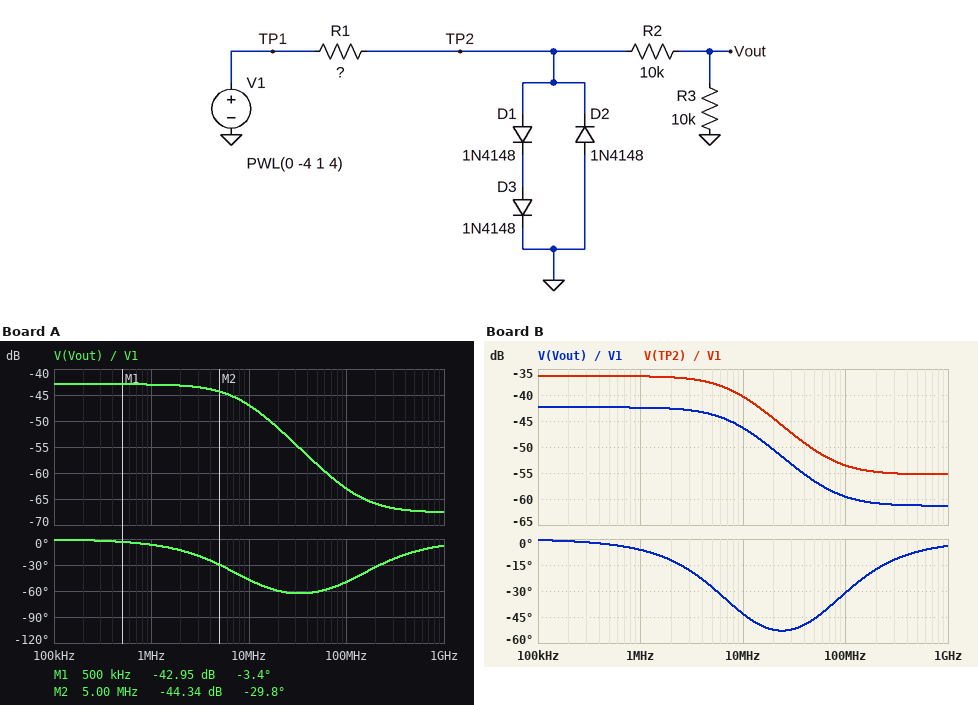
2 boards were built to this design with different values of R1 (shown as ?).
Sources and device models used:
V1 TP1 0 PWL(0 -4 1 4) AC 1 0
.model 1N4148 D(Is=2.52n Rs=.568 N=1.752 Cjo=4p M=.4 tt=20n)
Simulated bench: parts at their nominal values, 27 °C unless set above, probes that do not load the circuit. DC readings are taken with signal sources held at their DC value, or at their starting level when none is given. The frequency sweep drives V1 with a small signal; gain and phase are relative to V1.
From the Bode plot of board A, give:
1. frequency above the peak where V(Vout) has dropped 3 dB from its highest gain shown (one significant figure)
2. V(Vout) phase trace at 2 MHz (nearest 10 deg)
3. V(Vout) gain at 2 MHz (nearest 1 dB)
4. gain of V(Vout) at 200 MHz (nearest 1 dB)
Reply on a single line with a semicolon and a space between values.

8 MHz; -10 deg; -43 dB; -66 dB
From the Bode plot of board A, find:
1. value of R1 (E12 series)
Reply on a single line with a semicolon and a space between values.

680 Ω
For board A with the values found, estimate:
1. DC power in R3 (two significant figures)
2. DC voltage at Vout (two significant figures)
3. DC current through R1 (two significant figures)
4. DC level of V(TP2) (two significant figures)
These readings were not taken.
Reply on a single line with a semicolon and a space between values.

11 µW; -330 mV; 4.9 mA; -660 mV
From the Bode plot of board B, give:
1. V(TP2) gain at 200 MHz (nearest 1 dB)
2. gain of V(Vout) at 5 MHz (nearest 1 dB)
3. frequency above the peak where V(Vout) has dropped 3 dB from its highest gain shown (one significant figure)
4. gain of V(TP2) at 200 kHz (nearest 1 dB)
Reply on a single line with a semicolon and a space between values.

-55 dB; -44 dB; 8 MHz; -36 dB
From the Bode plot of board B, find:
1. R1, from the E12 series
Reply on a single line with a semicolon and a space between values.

330 Ω
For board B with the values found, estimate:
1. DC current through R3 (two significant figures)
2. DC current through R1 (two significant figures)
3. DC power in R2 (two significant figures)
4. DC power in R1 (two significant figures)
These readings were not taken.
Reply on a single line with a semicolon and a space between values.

35 µA; 10 mA; 12 µW; 33 mW
